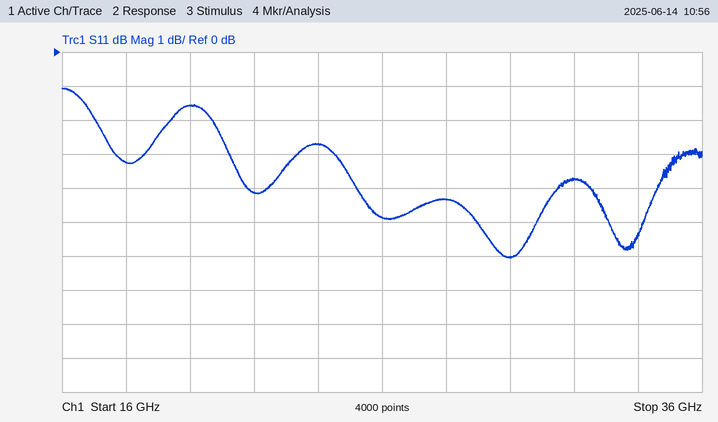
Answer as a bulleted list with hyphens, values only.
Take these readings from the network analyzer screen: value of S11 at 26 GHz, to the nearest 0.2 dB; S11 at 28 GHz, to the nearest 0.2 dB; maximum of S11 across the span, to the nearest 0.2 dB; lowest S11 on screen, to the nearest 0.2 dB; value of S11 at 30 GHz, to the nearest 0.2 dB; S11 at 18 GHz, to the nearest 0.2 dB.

- -4.8 dB
- -4.4 dB
- -1.0 dB
- -6.0 dB
- -6.0 dB
- -3.2 dB
